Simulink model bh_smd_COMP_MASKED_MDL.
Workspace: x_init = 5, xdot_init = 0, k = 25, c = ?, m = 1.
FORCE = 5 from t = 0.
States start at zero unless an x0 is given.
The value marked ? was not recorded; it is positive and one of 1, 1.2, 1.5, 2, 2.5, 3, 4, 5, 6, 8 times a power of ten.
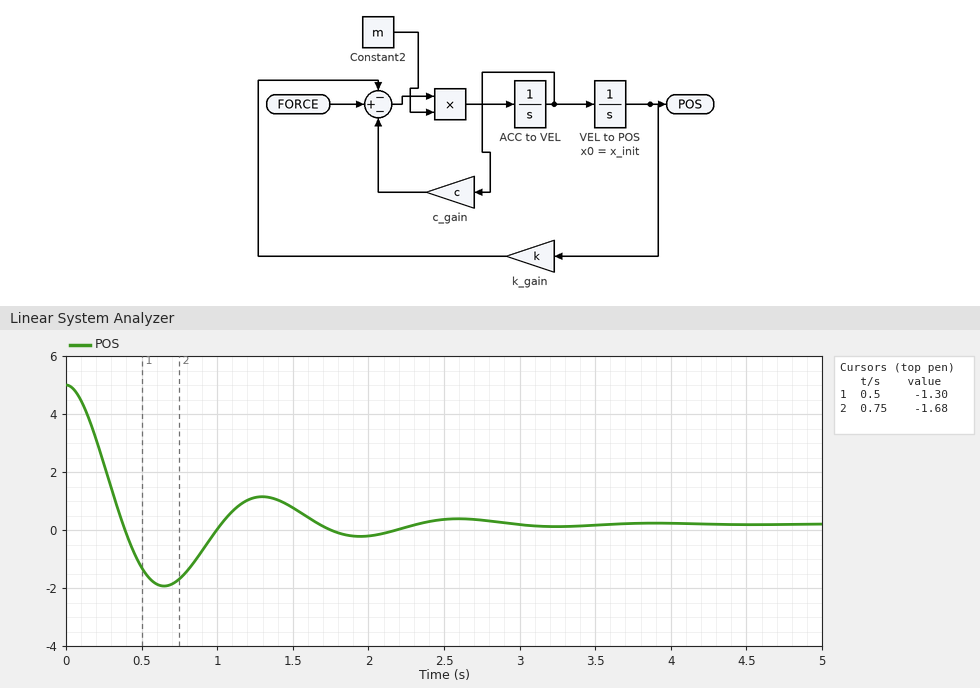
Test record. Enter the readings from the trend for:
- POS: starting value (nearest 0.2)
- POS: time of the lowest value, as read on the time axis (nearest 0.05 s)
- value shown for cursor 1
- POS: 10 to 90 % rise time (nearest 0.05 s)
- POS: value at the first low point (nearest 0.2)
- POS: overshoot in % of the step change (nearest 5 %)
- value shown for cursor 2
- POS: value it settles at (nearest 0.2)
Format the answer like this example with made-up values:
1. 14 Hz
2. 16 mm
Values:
1. 5.0
2. 0.65 s
3. -1.30
4. 0.25 s
5. -2.0
6. 45 %
7. -1.68
8. 0.2
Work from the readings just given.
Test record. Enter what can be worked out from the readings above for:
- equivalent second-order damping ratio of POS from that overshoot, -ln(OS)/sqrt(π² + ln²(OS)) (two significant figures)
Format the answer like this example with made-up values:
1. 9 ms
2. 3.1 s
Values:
1. 0.25
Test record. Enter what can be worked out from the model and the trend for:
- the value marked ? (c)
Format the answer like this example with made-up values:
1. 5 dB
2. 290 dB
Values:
1. 2.5
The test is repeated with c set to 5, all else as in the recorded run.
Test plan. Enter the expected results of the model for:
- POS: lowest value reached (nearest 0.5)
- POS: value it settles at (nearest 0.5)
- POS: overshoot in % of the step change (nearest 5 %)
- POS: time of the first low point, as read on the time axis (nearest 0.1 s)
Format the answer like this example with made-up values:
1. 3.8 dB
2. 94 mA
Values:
1. -0.5
2. 0.0
3. 15 %
4. 0.7 s
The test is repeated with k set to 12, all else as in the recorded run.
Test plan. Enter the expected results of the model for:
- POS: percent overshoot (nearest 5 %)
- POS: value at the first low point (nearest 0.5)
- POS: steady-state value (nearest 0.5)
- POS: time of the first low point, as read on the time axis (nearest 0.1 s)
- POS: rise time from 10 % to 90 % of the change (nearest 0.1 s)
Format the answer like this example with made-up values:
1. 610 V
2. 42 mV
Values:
1. 30 %
2. -1.0
3. 0.5
4. 1.0 s
5. 0.4 s
